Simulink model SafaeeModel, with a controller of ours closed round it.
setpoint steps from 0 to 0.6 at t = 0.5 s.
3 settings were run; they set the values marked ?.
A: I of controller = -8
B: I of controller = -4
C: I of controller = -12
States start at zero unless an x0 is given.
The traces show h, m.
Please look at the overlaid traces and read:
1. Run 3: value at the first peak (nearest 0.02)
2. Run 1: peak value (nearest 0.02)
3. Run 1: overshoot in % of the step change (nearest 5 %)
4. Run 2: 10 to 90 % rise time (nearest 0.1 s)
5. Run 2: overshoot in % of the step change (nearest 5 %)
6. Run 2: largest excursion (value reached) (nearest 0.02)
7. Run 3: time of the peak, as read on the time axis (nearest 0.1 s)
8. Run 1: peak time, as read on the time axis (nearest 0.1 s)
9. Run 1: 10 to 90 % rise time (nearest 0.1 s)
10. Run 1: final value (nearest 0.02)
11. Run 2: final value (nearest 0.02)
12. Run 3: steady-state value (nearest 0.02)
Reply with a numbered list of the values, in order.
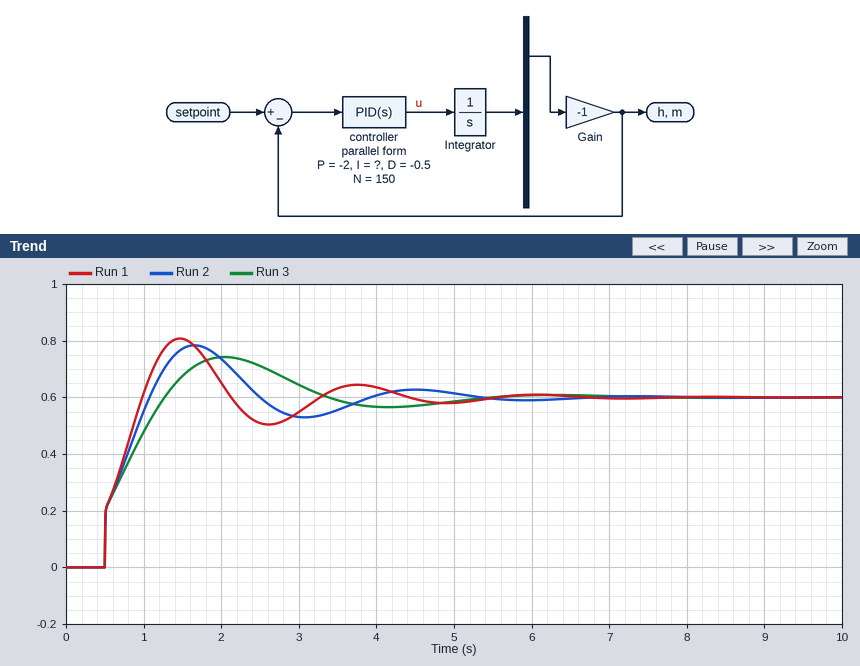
1. 0.74
2. 0.80
3. 35 %
4. 0.5 s
5. 30 %
6. 0.78
7. 2.0 s
8. 1.5 s
9. 0.4 s
10. 0.60
11. 0.60
12. 0.60
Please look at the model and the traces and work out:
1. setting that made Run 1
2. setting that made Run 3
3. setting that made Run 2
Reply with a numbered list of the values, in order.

1. C
2. B
3. A
